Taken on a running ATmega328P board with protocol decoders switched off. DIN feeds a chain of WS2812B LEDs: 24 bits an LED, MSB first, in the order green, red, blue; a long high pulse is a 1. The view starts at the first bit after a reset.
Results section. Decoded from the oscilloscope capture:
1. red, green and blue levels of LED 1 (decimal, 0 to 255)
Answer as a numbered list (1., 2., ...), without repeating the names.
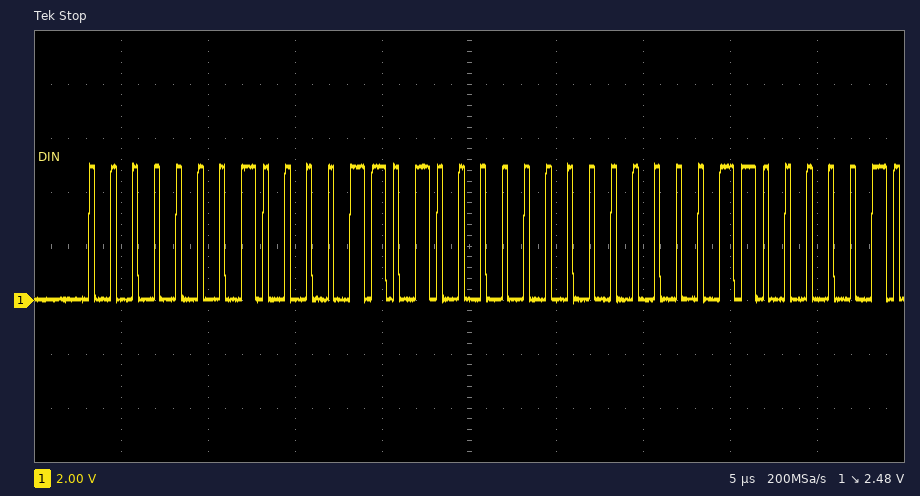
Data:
1. 13, 1, 0
